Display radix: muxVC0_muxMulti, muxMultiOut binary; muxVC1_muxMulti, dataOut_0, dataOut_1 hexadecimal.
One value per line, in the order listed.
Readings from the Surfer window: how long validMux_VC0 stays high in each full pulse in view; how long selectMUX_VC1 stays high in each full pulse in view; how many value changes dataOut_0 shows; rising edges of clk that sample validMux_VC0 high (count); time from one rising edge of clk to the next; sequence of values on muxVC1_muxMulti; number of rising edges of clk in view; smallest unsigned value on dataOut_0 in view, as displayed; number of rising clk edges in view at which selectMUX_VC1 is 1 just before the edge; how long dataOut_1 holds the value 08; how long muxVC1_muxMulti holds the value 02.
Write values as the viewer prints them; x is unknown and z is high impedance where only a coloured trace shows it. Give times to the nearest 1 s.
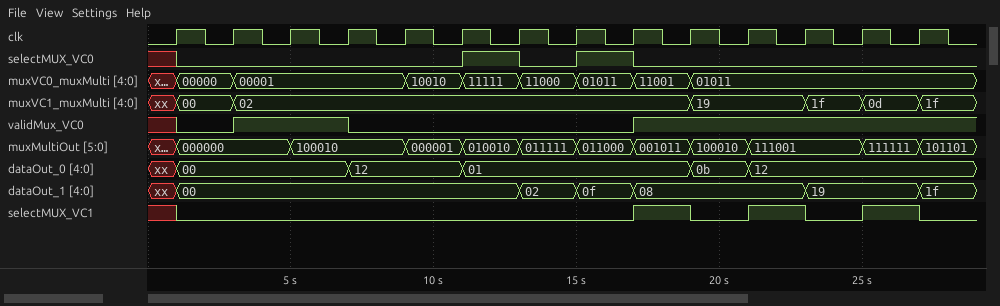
4 s
2 s, 2 s, 2 s
5
7
2 s
xx, 00, 02, 19, 1f, 0d, 1f
14
00
3
6 s
16 s
